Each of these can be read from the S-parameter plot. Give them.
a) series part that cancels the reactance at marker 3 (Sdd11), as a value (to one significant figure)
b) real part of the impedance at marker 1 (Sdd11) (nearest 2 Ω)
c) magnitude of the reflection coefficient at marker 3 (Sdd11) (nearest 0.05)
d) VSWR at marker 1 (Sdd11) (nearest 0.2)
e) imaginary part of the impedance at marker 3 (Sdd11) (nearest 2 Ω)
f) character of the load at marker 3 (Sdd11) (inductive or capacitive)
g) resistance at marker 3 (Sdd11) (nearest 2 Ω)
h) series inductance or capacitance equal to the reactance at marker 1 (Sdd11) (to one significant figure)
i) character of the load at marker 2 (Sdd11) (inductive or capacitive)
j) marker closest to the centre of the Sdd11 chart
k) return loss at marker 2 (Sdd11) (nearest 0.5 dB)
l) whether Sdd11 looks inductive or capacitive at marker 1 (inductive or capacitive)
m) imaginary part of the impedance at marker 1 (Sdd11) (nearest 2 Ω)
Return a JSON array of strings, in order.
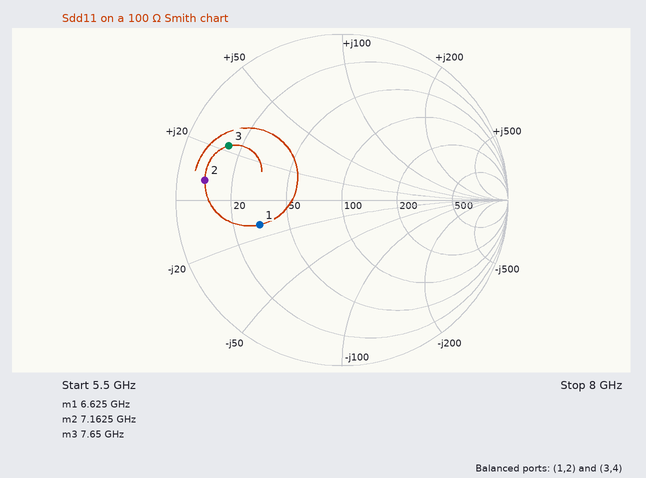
["900 fF", "32 Ω", "0.75", "3.2", "+22 Ω", "inductive", "14 Ω", "2 pF", "inductive", "marker 1", "1.5 dB", "capacitive", "-14 Ω"]
